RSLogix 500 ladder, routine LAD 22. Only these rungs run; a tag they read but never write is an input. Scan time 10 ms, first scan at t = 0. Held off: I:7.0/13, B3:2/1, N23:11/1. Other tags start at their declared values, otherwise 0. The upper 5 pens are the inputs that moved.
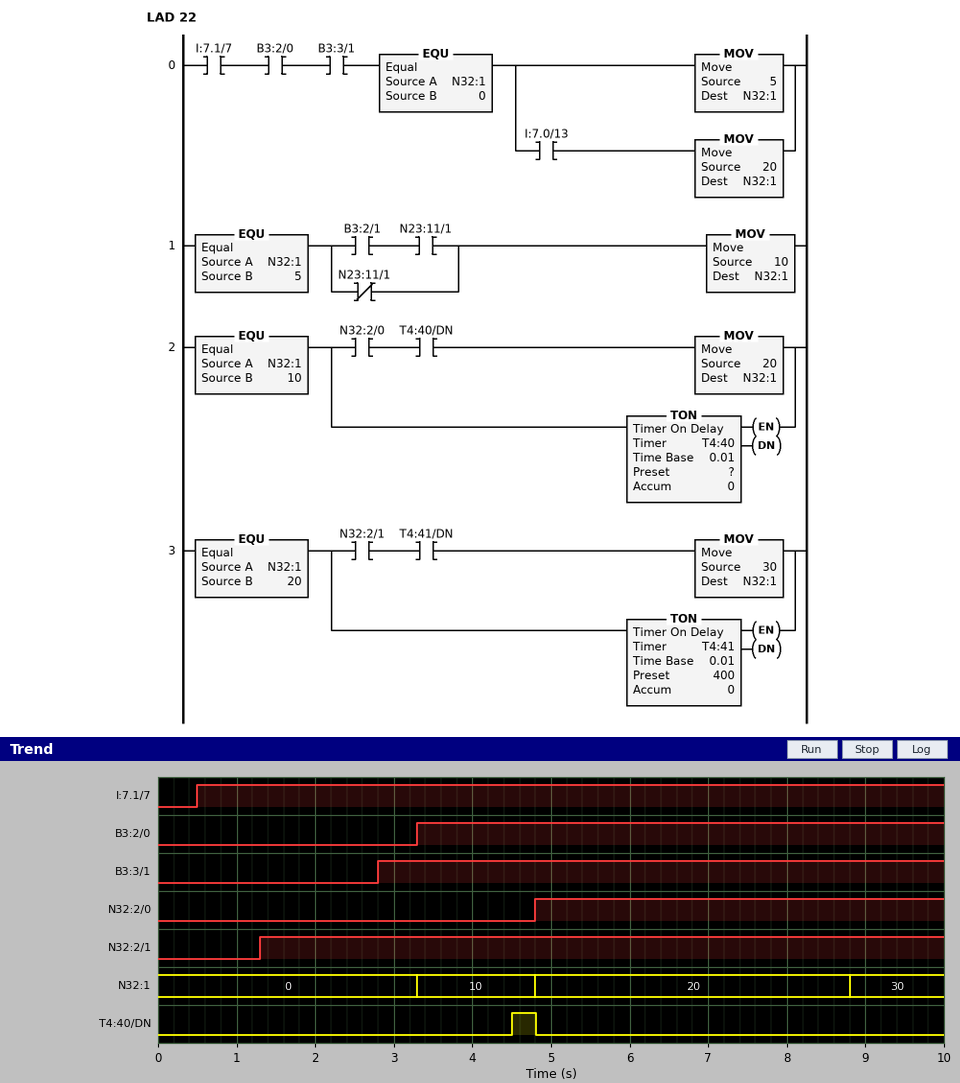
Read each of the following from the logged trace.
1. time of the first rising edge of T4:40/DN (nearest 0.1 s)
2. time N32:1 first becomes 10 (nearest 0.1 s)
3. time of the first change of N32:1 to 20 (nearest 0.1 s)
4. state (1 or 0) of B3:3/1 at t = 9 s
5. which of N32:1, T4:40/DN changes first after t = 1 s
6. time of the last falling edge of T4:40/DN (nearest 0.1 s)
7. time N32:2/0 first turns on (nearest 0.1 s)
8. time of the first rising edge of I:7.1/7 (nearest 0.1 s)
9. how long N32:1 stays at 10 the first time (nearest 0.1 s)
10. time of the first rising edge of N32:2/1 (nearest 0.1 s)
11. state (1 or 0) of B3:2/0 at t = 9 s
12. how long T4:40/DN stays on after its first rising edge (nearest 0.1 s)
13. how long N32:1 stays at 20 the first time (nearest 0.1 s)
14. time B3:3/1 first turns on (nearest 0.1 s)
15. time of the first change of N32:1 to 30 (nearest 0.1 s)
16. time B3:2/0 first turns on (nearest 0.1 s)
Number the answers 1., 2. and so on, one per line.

1. 4.5 s
2. 3.3 s
3. 4.8 s
4. 1
5. N32:1
6. 4.8 s
7. 4.8 s
8. 0.5 s
9. 1.5 s
10. 1.3 s
11. 1
12. 0.3 s
13. 4.0 s
14. 2.8 s
15. 8.8 s
16. 3.3 s
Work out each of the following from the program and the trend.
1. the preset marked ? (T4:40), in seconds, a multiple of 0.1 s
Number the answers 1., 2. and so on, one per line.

1. 1.2 s
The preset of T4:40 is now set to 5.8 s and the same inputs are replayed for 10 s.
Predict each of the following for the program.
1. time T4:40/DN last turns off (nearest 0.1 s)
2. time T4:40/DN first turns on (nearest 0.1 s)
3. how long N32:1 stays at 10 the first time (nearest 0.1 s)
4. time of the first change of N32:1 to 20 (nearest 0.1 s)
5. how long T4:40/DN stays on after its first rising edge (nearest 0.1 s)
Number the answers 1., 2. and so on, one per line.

1. 9.1 s
2. 9.1 s
3. 5.8 s
4. 9.1 s
5. 0.0 s
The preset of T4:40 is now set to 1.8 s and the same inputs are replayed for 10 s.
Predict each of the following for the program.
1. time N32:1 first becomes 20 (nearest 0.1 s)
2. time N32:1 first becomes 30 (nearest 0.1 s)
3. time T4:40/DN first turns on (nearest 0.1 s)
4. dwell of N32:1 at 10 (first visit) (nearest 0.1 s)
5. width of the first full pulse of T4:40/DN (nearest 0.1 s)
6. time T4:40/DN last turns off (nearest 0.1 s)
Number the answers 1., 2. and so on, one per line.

1. 5.1 s
2. 9.1 s
3. 5.1 s
4. 1.8 s
5. 0.0 s
6. 5.1 s
